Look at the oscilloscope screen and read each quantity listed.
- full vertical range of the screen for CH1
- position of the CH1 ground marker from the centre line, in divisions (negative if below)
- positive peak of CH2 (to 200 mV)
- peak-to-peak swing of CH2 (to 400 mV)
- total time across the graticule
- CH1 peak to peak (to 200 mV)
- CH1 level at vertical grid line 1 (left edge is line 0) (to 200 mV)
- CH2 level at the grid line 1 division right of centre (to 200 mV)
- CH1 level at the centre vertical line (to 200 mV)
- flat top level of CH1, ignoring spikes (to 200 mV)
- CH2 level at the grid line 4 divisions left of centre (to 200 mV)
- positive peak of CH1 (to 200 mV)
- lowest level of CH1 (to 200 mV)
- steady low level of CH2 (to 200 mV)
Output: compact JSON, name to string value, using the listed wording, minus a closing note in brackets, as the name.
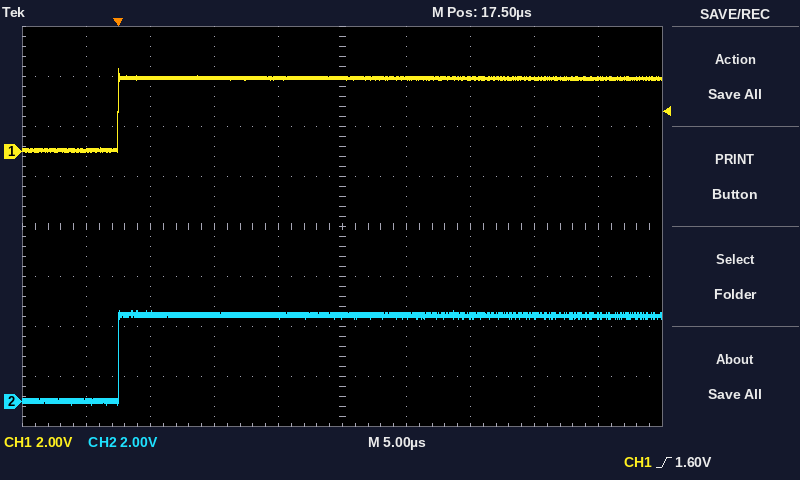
{"full vertical range of the screen for CH1": "16 V", "position of the CH1 ground marker from the centre line, in divisions": "+1.5 div", "positive peak of CH2": "3.6 V", "peak-to-peak swing of CH2": "3.6 V", "total time across the graticule": "50 µs", "CH1 peak to peak": "3.4 V", "CH1 level at vertical grid line 1 (left edge is line 0)": "0.0 V", "CH2 level at the grid line 1 division right of centre": "3.4 V", "CH1 level at the centre vertical line": "3.0 V", "flat top level of CH1, ignoring spikes": "3.0 V", "CH2 level at the grid line 4 divisions left of centre": "0.0 V", "positive peak of CH1": "3.4 V", "lowest level of CH1": "0.0 V", "steady low level of CH2": "0.0 V"}
